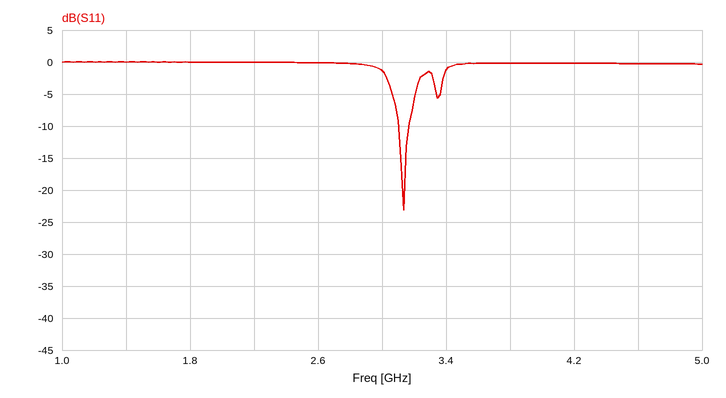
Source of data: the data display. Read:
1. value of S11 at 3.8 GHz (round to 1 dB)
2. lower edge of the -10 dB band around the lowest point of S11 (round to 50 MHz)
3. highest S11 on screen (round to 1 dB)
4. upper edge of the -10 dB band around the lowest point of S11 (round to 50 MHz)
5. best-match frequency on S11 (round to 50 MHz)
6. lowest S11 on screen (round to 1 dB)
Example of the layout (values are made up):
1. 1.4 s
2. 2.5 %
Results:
1. 0 dB
2. 3.10 GHz
3. 0 dB
4. 3.15 GHz
5. 3.15 GHz
6. -23 dB
